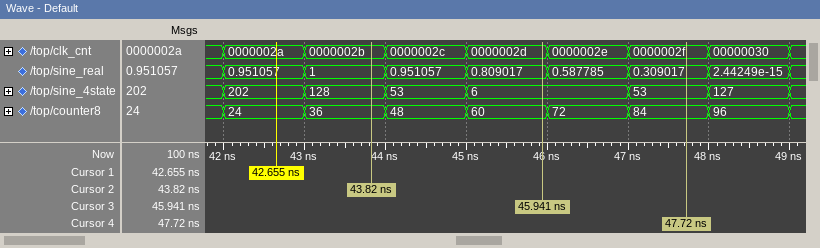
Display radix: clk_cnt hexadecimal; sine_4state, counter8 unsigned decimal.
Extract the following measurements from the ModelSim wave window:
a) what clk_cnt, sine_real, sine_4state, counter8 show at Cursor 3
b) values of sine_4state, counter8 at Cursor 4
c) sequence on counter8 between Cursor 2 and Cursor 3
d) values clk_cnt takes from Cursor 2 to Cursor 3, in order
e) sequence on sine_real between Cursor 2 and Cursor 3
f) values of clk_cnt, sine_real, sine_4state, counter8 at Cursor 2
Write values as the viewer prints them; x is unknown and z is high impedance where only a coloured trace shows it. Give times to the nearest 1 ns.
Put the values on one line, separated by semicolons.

clk_cnt=0000002d, sine_real=0.809017, sine_4state=6, counter8=60; sine_4state=53, counter8=84; 36, 48, 60; 0000002b, 0000002c, 0000002d; 1, 0.951057, 0.809017; clk_cnt=0000002b, sine_real=1, sine_4state=128, counter8=36
